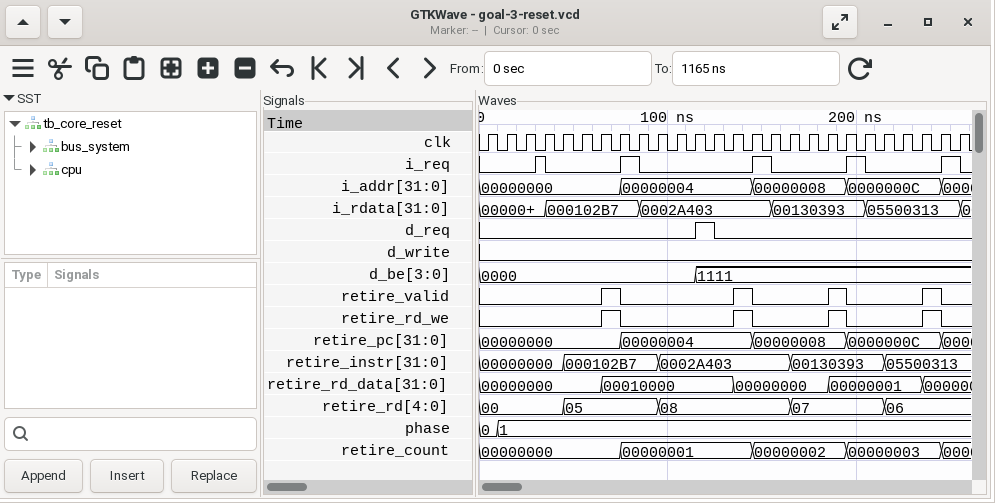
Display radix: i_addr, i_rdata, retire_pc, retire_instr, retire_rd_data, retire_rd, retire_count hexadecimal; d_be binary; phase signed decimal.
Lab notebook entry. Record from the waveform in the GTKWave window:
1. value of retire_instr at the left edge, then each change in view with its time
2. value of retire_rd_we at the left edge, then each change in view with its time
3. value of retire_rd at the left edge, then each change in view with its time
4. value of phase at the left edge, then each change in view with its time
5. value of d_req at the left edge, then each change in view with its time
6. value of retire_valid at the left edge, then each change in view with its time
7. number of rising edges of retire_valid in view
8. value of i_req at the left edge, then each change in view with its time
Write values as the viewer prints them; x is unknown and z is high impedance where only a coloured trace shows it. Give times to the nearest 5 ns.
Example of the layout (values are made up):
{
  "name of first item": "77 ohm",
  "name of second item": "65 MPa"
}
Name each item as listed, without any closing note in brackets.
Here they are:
{
  "value of retire_instr at the left edge, then each change in view with its time": "00000000, 000102B7 at 45 ns, 0002A403 at 95 ns, 00130393 at 165 ns, 05500313 at 215 ns",
  "value of retire_rd_we at the left edge, then each change in view with its time": "0, 1 at 65 ns, 0 at 75 ns, 1 at 135 ns, 0 at 145 ns, 1 at 185 ns, 0 at 195 ns, 1 at 235 ns, 0 at 245 ns",
  "value of retire_rd at the left edge, then each change in view with its time": "00, 05 at 45 ns, 08 at 95 ns, 07 at 165 ns, 06 at 215 ns",
  "value of phase at the left edge, then each change in view with its time": "0, 1 at 10 ns",
  "value of d_req at the left edge, then each change in view with its time": "0, 1 at 115 ns, 0 at 125 ns",
  "value of retire_valid at the left edge, then each change in view with its time": "0, 1 at 65 ns, 0 at 75 ns, 1 at 135 ns, 0 at 145 ns, 1 at 185 ns, 0 at 195 ns, 1 at 235 ns, 0 at 245 ns",
  "number of rising edges of retire_valid in view": "4",
  "value of i_req at the left edge, then each change in view with its time": "0, 1 at 30 ns, 0 at 35 ns, 1 at 75 ns, 0 at 85 ns, 1 at 145 ns, 0 at 155 ns, 1 at 195 ns, 0 at 205 ns, 1 at 245 ns, 0 at 255 ns"
}
